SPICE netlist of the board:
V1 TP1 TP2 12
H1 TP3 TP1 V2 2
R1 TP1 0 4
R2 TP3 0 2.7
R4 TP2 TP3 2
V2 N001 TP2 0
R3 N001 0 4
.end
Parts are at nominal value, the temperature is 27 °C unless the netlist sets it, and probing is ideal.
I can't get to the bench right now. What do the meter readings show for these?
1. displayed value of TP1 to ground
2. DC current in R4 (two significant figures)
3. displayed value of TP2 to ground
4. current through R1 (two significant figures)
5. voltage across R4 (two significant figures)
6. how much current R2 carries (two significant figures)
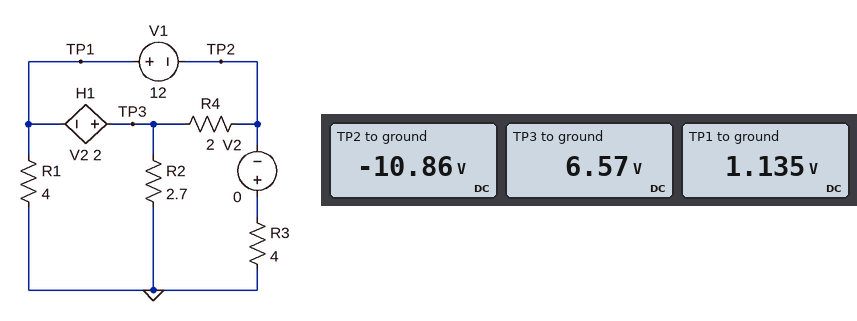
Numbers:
1.135 V
8.7 A
-10.86 V
280 mA
17 V
2.4 A
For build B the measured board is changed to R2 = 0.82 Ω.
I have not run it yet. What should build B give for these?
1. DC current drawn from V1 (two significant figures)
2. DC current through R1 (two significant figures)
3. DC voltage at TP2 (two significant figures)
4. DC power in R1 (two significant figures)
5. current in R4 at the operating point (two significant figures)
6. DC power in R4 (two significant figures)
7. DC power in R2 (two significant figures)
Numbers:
14 A
970 mA
-16 V
3.8 W
10 A
200 W
20 W
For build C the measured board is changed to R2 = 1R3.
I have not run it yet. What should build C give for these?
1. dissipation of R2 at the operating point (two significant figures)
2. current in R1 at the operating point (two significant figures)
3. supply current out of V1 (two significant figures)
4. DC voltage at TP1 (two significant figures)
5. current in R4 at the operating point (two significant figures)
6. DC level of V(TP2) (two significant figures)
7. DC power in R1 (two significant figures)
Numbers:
20 W
460 mA
13 A
-1.8 V
9.5 A
-14 V
830 mW
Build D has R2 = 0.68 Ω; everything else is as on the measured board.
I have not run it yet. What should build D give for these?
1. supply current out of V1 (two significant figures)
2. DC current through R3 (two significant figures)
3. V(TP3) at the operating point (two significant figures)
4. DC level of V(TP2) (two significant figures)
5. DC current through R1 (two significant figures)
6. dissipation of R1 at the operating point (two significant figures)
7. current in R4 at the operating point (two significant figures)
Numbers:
14 A
4.2 A
3.6 V
-17 V
1.2 A
5.6 W
10 A
